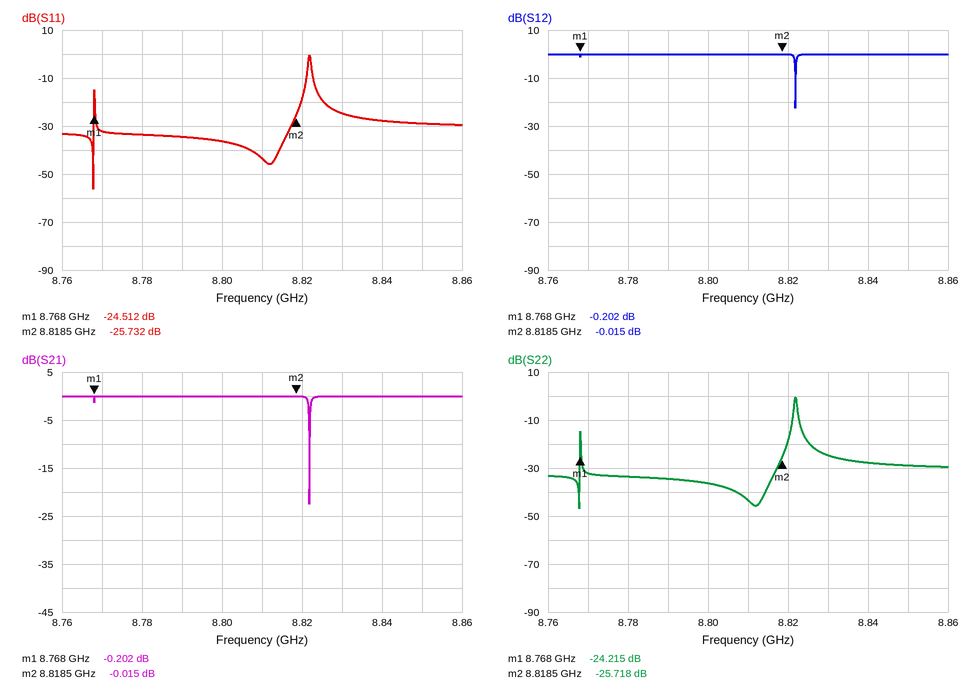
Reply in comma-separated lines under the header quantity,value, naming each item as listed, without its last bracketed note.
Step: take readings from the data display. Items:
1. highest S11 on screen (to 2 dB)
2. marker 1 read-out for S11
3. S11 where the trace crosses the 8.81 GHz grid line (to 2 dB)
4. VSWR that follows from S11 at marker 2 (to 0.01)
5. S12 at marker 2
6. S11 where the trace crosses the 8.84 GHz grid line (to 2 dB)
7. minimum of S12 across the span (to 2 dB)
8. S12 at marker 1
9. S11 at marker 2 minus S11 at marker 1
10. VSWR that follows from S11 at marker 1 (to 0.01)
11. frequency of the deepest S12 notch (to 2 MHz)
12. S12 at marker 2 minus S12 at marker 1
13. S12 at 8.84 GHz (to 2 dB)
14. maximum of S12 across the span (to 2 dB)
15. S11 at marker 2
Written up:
quantity,value
highest S11 on screen,0 dB
marker 1 read-out for S11,-24.512 dB
S11 where the trace crosses the 8.81 GHz grid line,-44 dB
VSWR that follows from S11 at marker 2,1.11
S12 at marker 2,-0.015 dB
S11 where the trace crosses the 8.84 GHz grid line,-28 dB
minimum of S12 across the span,-22 dB
S12 at marker 1,-0.202 dB
S11 at marker 2 minus S11 at marker 1,-1.220 dB
VSWR that follows from S11 at marker 1,1.13
frequency of the deepest S12 notch,8.822 GHz
S12 at marker 2 minus S12 at marker 1,0.187 dB
S12 at 8.84 GHz,0 dB
maximum of S12 across the span,0 dB
S11 at marker 2,-25.732 dB
